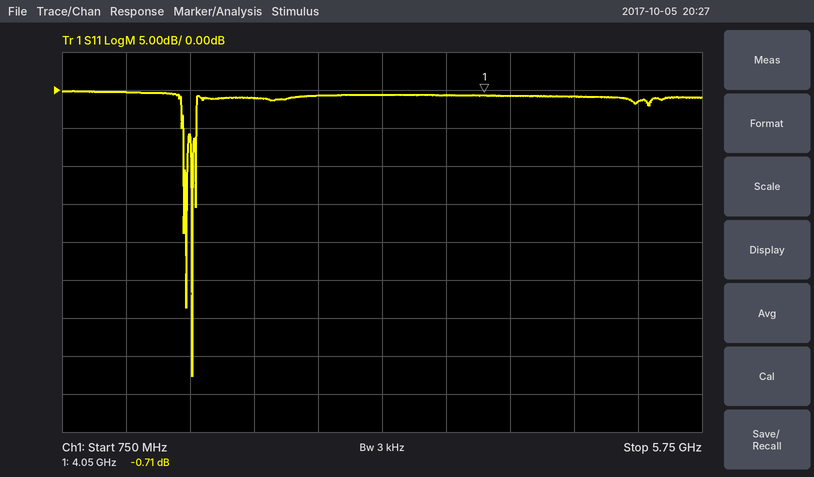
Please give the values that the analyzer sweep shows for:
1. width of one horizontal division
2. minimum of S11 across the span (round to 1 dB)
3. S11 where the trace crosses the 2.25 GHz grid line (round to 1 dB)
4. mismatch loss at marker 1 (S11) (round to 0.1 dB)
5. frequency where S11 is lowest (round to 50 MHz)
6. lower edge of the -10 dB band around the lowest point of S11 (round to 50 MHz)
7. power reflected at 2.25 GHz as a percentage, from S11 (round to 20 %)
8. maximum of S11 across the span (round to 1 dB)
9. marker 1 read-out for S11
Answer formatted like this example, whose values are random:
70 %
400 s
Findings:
500 MHz
-38 dB
-1 dB
8.2 dB
1.75 GHz
1.75 GHz
80 %
0 dB
-0.71 dB
